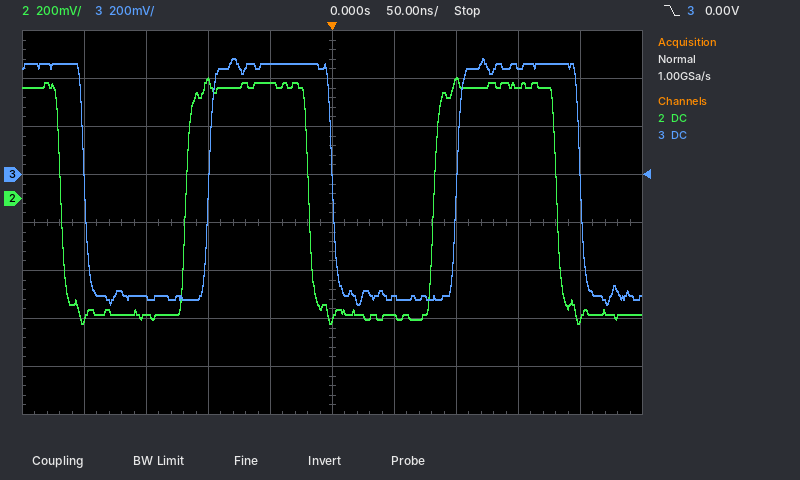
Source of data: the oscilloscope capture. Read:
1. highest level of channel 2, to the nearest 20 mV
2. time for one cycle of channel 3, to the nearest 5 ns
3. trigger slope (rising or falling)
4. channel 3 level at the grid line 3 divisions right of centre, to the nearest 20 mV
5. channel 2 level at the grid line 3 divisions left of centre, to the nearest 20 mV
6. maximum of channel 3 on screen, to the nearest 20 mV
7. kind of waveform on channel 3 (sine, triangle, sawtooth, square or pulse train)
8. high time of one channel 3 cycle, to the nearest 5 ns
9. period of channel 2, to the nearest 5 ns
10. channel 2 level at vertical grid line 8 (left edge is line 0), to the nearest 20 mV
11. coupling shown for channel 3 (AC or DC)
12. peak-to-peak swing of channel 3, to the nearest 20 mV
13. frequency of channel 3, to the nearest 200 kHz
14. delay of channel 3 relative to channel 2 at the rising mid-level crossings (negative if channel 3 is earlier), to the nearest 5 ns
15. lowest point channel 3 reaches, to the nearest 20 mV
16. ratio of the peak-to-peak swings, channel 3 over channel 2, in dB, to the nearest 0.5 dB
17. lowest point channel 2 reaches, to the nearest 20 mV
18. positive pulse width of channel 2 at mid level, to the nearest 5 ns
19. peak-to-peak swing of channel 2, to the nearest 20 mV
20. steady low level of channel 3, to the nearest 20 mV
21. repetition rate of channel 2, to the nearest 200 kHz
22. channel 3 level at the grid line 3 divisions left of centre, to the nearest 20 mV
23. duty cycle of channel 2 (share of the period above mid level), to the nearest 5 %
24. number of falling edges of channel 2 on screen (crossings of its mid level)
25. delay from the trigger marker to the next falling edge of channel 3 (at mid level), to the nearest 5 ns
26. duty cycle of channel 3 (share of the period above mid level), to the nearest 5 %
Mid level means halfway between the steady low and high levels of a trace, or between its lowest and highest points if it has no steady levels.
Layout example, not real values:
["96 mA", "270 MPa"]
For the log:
["500 mV", "200 ns", "falling", "460 mV", "-480 mV", "480 mV", "square", "100 ns", "200 ns", "460 mV", "DC", "1.02 V", "5.0 MHz", "+20 ns", "-540 mV", "0.0 dB", "-520 mV", "100 ns", "1.02 V", "-500 mV", "5.0 MHz", "-520 mV", "50 %", "3", "200 ns", "50 %"]
